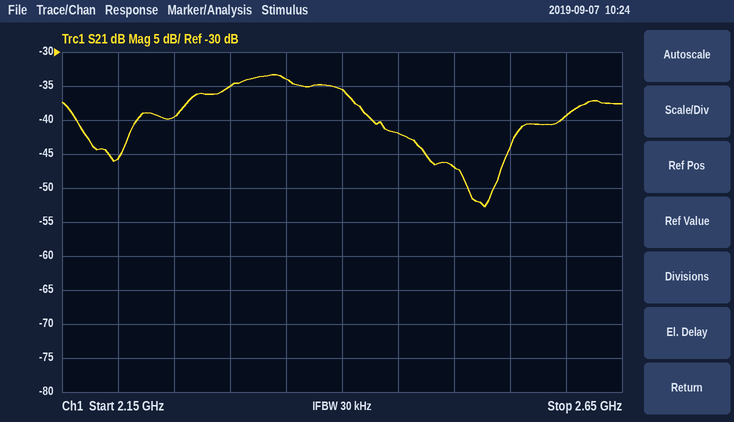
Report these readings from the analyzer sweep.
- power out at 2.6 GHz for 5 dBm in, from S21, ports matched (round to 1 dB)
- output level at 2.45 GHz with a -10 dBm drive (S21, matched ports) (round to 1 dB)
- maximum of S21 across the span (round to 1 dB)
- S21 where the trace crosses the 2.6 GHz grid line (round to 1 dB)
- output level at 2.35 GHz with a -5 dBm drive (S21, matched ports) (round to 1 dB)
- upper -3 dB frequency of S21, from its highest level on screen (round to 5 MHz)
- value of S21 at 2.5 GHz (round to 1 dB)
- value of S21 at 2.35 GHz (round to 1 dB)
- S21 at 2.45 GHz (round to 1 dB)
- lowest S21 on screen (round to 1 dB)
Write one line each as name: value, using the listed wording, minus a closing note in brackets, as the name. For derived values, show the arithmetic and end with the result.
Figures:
power out at 2.6 GHz for 5 dBm in, from S21, ports matched: 5 dBm + (-39 dB) = -34 dBm
output level at 2.45 GHz with a -10 dBm drive (S21, matched ports): -10 dBm + (-42 dB) = -52 dBm
maximum of S21 across the span: -33 dB
S21 where the trace crosses the 2.6 GHz grid line: -39 dB
output level at 2.35 GHz with a -5 dBm drive (S21, matched ports): -5 dBm + (-34 dB) = -39 dBm
upper -3 dB frequency of S21, from its highest level on screen: 2.405 GHz
value of S21 at 2.5 GHz: -47 dB
value of S21 at 2.35 GHz: -34 dB
S21 at 2.45 GHz: -42 dB
lowest S21 on screen: -53 dB
